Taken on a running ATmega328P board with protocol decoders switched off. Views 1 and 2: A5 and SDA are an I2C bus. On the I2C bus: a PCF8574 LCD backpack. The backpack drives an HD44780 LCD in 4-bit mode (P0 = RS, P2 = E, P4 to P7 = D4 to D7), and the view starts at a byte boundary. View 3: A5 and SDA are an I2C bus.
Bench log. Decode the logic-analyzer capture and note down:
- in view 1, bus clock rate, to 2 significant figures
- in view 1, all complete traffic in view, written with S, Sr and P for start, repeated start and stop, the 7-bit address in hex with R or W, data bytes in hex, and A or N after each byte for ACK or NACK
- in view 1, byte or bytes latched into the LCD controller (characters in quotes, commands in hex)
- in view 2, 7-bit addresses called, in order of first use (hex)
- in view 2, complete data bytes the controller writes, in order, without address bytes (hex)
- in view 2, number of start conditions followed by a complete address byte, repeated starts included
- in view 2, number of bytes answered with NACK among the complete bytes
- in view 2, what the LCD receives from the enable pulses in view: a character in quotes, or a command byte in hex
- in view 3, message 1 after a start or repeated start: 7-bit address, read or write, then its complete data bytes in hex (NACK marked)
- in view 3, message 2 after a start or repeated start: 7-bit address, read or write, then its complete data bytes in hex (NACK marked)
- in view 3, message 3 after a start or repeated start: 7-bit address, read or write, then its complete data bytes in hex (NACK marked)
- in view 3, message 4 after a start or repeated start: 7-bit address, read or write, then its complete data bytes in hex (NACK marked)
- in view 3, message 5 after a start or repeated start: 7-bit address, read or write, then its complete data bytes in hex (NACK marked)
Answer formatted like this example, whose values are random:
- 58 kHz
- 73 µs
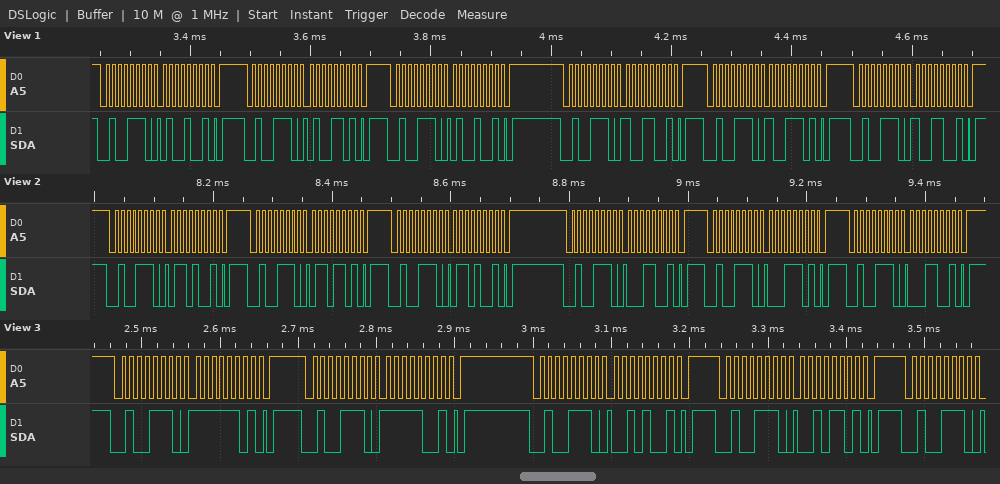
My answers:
- 100 kHz
- S 27W A 49 A P S 27W A 4D A P S 27W A 49 A P S 27W A 99 A P S 27W A 9D A P S 27W A 99 A P
- 'I'
- 0x27
- 69 6D 69 19 1D 19
- 6
- 0
- 'a'
- 0x27 write: FD
- 0x27 write: F9
- 0x27 write: 29
- 0x27 write: 2D
- 0x27 write
